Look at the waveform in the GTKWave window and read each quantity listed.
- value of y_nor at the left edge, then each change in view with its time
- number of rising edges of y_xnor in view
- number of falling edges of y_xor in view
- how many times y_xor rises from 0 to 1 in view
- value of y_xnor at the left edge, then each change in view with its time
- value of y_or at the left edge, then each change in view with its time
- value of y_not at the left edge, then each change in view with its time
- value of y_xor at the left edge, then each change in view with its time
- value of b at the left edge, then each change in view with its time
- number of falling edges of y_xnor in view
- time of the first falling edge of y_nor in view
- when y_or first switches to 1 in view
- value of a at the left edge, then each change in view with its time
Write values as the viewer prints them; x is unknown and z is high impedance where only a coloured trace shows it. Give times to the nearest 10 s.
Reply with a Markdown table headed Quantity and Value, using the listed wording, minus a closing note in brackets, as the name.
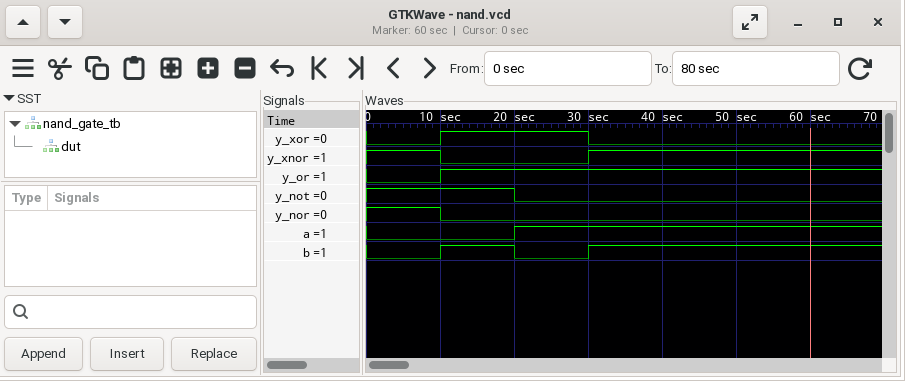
| Quantity | Value |
|---|---|
| value of y_nor at the left edge, then each change in view with its time | 1, 0 at 10 s |
| number of rising edges of y_xnor in view | 1 |
| number of falling edges of y_xor in view | 1 |
| how many times y_xor rises from 0 to 1 in view | 1 |
| value of y_xnor at the left edge, then each change in view with its time | 1, 0 at 10 s, 1 at 30 s |
| value of y_or at the left edge, then each change in view with its time | 0, 1 at 10 s |
| value of y_not at the left edge, then each change in view with its time | 1, 0 at 20 s |
| value of y_xor at the left edge, then each change in view with its time | 0, 1 at 10 s, 0 at 30 s |
| value of b at the left edge, then each change in view with its time | 0, 1 at 10 s, 0 at 20 s, 1 at 30 s |
| number of falling edges of y_xnor in view | 1 |
| time of the first falling edge of y_nor in view | 10 s |
| when y_or first switches to 1 in view | 10 s |
| value of a at the left edge, then each change in view with its time | 0, 1 at 20 s |
